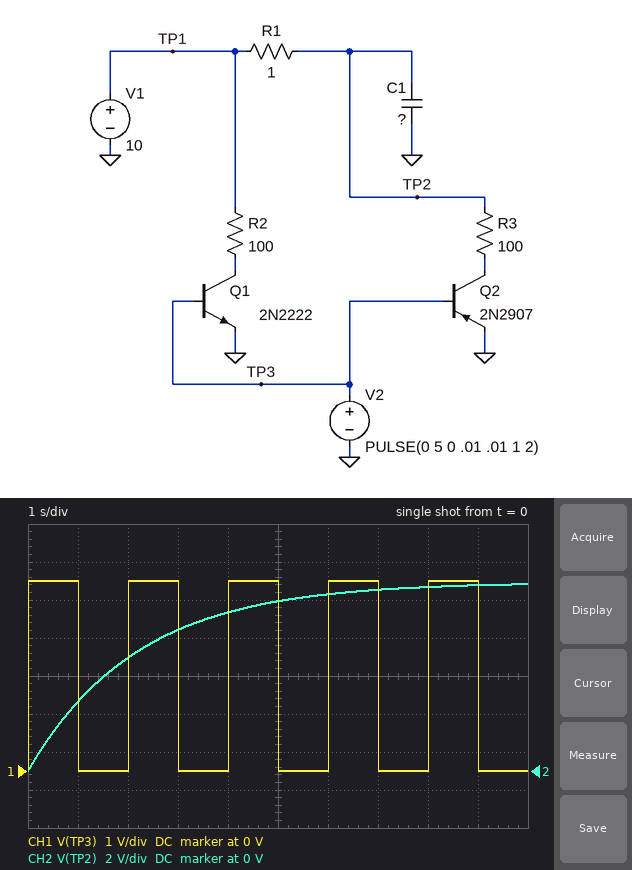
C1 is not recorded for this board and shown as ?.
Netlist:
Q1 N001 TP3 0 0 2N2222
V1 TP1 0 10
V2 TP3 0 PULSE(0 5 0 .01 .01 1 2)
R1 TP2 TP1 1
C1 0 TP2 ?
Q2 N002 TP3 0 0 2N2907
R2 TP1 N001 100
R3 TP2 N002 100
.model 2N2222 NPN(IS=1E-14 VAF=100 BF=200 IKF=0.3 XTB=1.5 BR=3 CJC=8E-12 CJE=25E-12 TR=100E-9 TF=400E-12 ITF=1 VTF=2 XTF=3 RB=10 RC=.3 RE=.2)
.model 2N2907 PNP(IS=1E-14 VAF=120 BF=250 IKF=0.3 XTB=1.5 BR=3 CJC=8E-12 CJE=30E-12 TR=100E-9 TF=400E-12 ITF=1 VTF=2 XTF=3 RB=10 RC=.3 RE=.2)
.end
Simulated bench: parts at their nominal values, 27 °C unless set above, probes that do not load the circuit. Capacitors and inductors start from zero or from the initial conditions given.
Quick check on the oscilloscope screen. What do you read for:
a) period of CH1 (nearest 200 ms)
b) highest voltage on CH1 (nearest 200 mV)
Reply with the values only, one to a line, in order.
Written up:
2.0 s
5.0 V
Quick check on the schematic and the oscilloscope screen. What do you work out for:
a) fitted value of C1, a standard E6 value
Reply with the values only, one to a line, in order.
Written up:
2.2 F
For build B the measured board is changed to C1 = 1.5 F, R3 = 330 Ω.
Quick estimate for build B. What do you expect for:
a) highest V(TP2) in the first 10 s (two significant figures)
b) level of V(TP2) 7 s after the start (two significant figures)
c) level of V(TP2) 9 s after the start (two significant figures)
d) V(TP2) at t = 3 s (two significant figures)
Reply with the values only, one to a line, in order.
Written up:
10 V
9.9 V
10 V
8.6 V
